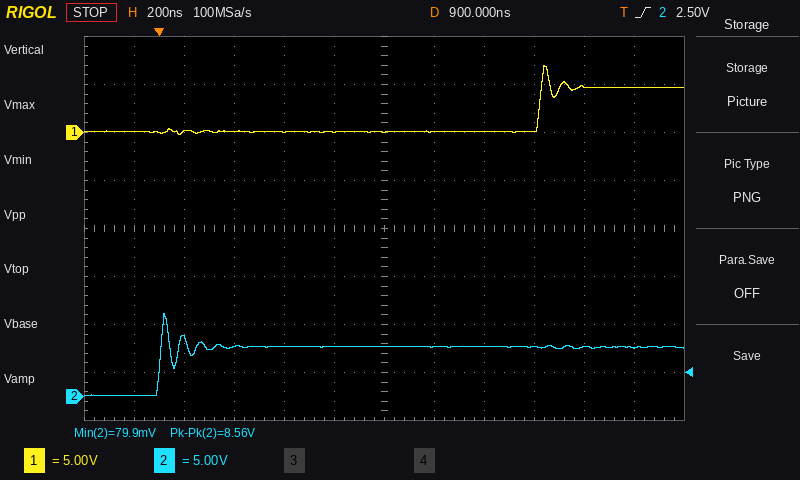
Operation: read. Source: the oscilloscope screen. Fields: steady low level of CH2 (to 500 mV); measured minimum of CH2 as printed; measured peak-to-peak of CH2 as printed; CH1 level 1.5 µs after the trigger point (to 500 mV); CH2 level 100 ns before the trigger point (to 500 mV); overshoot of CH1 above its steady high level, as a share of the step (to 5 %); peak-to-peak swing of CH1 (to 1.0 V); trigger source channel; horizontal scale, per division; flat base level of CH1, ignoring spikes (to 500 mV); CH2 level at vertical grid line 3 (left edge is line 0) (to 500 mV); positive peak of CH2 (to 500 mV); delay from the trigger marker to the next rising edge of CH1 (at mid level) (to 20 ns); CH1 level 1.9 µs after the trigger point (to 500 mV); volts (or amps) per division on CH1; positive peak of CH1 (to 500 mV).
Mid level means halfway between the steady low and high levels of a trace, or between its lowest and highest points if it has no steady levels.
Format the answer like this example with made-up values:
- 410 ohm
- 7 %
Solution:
- 0.0 V
- 79.9 mV
- 8.56 V
- 500 mV
- 0.0 V
- 50 %
- 7.0 V
- CH2
- 200 ns
- 0.0 V
- 5.0 V
- 8.5 V
- 1.52 µs
- 4.5 V
- 5 V
- 7.0 V
